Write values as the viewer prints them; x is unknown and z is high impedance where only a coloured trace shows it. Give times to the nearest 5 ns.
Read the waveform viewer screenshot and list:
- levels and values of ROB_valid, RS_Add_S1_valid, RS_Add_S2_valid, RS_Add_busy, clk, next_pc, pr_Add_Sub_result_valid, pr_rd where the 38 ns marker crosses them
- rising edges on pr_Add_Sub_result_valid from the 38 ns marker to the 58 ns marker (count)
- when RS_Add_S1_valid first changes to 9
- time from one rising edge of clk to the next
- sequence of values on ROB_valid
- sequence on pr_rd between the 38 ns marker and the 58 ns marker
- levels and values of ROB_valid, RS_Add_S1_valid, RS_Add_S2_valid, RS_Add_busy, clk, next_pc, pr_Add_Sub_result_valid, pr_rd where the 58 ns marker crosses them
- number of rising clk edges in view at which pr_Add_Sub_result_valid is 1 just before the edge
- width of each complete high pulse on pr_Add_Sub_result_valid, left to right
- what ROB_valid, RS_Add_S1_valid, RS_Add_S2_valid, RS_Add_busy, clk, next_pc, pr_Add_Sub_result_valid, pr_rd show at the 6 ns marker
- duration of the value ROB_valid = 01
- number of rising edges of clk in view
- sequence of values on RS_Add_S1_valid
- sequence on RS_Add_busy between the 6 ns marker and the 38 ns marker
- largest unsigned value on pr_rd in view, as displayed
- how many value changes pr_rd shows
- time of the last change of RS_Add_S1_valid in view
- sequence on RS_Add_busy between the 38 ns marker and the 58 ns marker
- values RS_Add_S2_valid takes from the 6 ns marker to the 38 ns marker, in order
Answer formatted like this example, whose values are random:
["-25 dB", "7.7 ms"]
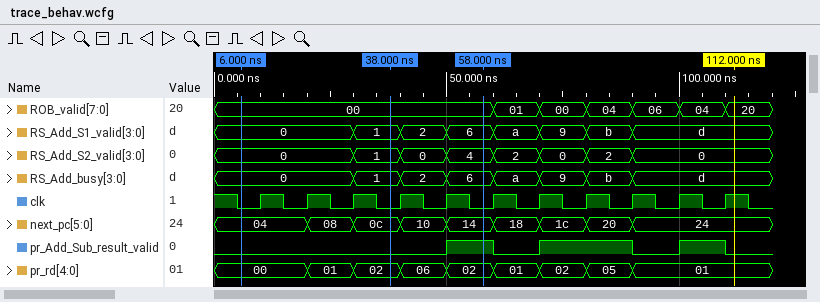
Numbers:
["ROB_valid=00, RS_Add_S1_valid=1, RS_Add_S2_valid=1, RS_Add_busy=1, clk=0, next_pc=0c, pr_Add_Sub_result_valid=0, pr_rd=02", "1", "70 ns", "10 ns", "00, 01, 00, 04, 06, 04, 20", "02, 06, 02", "ROB_valid=00, RS_Add_S1_valid=6, RS_Add_S2_valid=4, RS_Add_busy=6, clk=0, next_pc=14, pr_Add_Sub_result_valid=1, pr_rd=02", "4", "10 ns, 20 ns, 10 ns", "ROB_valid=00, RS_Add_S1_valid=0, RS_Add_S2_valid=0, RS_Add_busy=0, clk=0, next_pc=04, pr_Add_Sub_result_valid=0, pr_rd=00", "10 ns", "11", "0, 1, 2, 6, a, 9, b, d", "0, 1", "06", "8", "90 ns", "1, 2, 6", "0, 1"]
